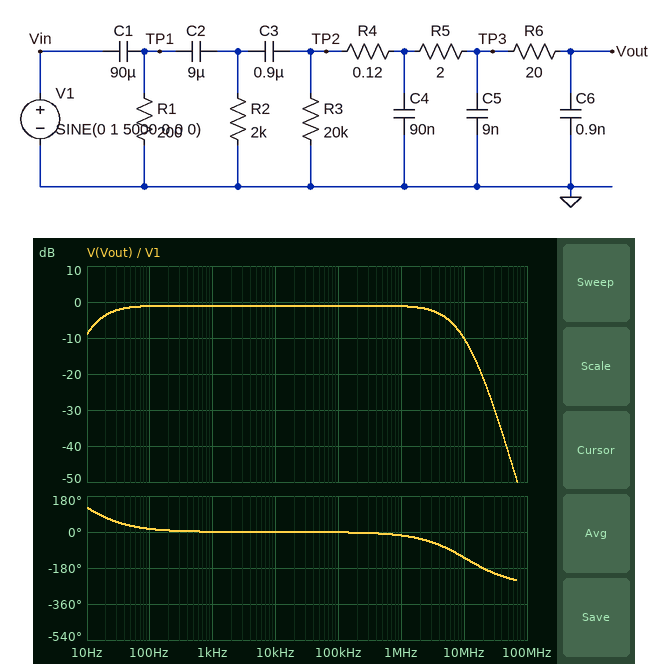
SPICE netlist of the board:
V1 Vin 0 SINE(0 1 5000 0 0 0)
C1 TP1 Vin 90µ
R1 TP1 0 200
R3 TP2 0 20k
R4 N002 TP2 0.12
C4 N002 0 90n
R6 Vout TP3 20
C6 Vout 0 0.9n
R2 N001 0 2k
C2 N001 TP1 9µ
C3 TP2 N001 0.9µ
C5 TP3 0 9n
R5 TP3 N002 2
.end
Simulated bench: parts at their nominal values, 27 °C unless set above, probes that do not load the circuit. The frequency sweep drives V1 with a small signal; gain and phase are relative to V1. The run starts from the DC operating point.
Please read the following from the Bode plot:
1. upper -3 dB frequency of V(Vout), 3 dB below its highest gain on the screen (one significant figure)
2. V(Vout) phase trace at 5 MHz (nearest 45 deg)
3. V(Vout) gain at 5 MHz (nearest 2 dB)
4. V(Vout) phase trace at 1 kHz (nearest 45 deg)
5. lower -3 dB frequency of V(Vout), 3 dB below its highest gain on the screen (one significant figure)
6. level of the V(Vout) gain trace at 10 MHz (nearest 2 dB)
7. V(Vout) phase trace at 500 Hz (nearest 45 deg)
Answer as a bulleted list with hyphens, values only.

- 5 MHz
- -90 deg
- -4 dB
- 0 deg
- 20 Hz
- -10 dB
- 0 deg
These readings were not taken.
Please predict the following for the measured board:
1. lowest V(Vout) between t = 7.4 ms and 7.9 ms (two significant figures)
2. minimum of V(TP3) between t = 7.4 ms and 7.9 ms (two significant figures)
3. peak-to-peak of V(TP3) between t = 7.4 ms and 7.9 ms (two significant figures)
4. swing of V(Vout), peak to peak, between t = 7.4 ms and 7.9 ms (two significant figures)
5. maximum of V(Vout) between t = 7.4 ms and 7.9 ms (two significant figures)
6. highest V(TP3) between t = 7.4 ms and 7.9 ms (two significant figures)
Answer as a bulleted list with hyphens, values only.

- -890 mV
- -890 mV
- 1.8 V
- 1.8 V
- 890 mV
- 890 mV
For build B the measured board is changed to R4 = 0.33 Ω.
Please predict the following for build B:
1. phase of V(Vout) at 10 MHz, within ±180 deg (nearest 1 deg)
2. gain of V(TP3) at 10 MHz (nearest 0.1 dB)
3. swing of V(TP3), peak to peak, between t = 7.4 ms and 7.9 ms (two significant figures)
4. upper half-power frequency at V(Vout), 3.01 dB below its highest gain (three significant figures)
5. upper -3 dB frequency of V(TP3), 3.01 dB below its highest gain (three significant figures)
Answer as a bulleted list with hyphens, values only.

- -155 deg
- -11.2 dB
- 1.8 V
- 3.47 MHz
- 4.00 MHz
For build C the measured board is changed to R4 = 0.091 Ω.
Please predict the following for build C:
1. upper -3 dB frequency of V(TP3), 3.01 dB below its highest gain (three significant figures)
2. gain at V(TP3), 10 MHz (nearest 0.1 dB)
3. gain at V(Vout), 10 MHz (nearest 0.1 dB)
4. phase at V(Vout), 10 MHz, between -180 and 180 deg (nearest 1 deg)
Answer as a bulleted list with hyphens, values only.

- 6.91 MHz
- -6.0 dB
- -9.6 dB
- -122 deg
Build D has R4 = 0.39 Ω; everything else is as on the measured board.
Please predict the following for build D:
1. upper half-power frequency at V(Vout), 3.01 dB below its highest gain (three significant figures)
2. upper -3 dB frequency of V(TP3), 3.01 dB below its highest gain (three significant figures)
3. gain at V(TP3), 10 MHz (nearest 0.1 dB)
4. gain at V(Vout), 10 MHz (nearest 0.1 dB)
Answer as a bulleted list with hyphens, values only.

- 3.18 MHz
- 3.58 MHz
- -12.3 dB
- -15.9 dB
